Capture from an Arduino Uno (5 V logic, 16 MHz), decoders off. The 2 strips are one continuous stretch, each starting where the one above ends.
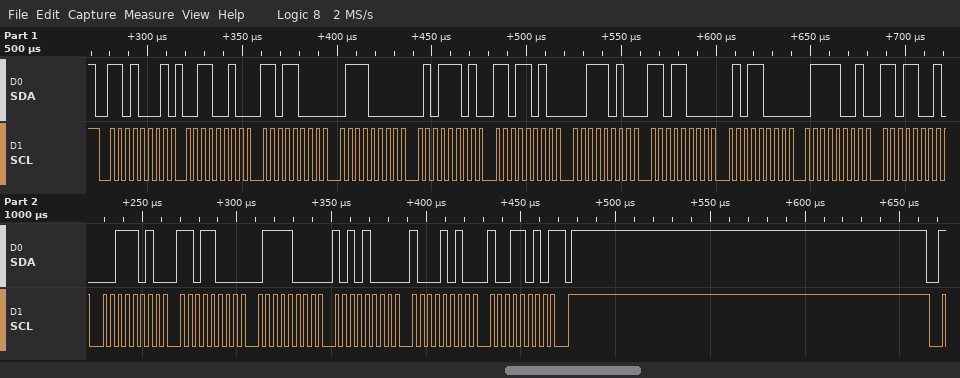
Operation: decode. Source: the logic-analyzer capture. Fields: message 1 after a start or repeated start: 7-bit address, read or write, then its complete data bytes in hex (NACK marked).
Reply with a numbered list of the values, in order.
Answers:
1. 0x68 read: 32 D8 70 5D DA 3A D8 58 79 D9 3A D8 78 A8 8A 9A NACK
